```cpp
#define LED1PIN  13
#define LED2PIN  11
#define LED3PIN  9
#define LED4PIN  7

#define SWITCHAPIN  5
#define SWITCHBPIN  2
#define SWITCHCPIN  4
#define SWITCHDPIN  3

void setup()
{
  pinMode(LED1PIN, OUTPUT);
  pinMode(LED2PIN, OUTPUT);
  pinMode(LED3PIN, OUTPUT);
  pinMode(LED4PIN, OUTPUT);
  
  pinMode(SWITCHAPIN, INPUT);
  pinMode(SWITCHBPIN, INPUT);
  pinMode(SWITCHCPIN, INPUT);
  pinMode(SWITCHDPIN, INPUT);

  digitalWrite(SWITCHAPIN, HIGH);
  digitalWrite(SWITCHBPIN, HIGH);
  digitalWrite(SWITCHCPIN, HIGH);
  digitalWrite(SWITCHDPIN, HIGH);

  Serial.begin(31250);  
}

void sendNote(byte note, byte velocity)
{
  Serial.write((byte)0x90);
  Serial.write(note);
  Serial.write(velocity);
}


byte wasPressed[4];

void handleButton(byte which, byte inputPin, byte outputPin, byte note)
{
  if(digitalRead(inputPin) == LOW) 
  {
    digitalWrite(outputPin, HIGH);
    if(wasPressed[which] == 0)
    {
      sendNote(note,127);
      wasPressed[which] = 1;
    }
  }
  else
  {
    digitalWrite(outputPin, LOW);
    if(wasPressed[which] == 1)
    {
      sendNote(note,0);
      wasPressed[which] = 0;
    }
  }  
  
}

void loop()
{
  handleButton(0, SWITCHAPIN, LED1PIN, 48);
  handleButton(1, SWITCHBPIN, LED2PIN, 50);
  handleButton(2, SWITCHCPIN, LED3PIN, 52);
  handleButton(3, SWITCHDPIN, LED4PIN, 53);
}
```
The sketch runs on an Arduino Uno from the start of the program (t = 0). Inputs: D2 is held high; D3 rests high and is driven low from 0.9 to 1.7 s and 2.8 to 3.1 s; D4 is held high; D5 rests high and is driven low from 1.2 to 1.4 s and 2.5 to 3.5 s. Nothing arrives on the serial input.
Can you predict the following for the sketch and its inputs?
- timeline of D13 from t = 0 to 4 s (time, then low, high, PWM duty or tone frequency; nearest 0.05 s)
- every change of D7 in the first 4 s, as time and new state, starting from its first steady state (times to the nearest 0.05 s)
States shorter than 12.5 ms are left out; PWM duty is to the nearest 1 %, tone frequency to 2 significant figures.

0 s low; 1.2 s high; 1.4 s low; 2.5 s high; 3.5 s low
0 s low; 0.9 s high; 1.7 s low; 2.8 s high; 3.1 s low
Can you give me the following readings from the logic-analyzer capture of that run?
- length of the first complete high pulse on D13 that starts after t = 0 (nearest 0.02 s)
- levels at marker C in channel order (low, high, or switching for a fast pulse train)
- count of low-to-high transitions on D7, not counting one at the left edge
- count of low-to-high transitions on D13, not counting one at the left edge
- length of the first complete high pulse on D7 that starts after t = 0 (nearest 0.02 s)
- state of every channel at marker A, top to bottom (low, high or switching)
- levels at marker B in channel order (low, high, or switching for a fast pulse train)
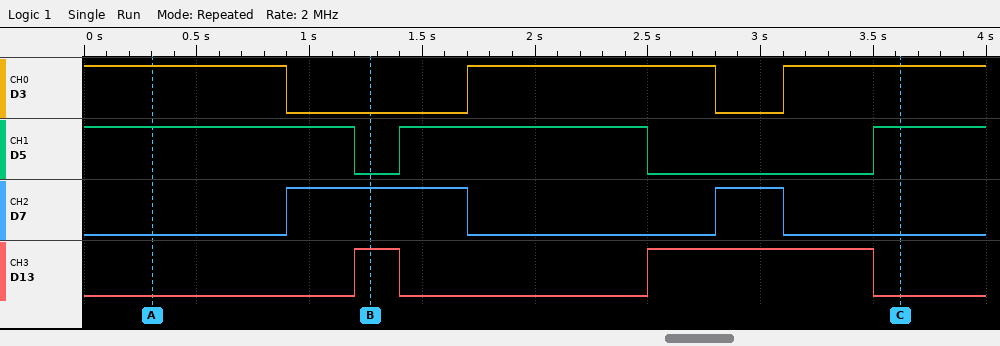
0.20 s
D3 high, D5 high, D7 low, D13 low
2
2
0.80 s
D3 high, D5 high, D7 low, D13 low
D3 low, D5 low, D7 high, D13 high
